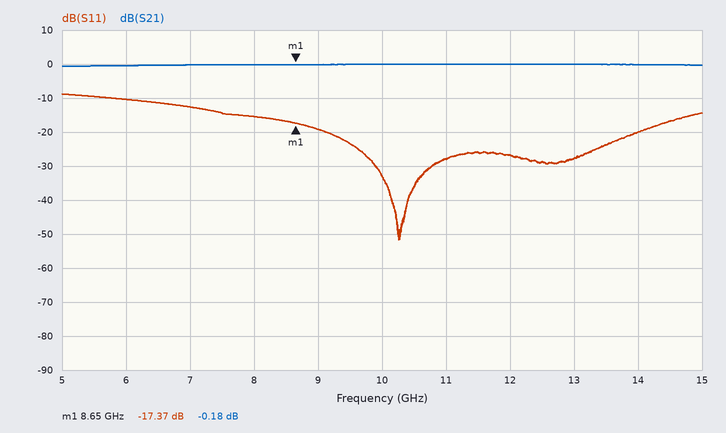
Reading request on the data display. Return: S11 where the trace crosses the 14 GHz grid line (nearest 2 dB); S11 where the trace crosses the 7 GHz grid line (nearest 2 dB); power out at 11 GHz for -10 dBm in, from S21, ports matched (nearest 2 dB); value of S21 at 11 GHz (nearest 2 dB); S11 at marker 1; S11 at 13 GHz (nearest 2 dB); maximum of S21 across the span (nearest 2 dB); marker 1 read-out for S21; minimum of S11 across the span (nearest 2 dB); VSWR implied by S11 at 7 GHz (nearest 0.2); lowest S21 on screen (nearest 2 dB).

-20 dB
-12 dB
-10 dBm
0 dB
-17.37 dB
-28 dB
0 dB
-0.18 dB
-52 dB
1.6
0 dB
